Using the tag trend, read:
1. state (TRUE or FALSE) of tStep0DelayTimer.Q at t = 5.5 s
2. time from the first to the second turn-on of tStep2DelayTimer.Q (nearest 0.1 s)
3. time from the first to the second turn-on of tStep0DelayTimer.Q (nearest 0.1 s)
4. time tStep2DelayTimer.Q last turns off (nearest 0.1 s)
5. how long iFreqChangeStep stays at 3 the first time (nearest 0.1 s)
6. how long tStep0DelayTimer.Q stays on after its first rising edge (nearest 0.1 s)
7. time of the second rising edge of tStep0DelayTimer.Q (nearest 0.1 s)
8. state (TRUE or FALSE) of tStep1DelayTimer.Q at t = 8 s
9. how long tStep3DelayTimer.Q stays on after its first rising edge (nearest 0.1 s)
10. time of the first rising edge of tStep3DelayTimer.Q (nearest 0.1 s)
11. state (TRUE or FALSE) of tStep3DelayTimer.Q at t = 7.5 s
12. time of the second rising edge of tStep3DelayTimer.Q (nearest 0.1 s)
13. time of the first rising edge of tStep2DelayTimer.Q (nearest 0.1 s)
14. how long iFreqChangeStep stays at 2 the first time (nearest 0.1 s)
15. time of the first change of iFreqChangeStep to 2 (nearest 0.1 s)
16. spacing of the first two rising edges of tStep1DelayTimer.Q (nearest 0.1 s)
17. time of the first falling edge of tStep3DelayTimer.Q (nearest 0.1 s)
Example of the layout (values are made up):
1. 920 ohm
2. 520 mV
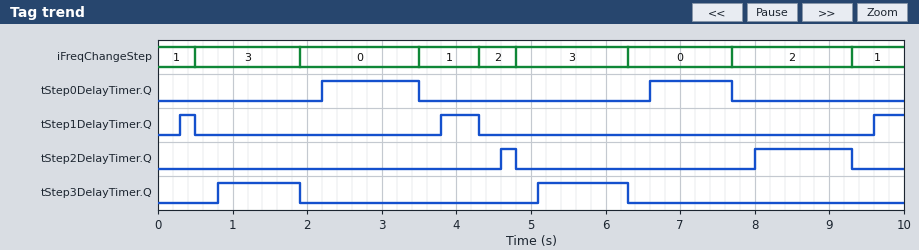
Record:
1. FALSE
2. 3.4 s
3. 4.4 s
4. 9.3 s
5. 1.4 s
6. 1.3 s
7. 6.6 s
8. FALSE
9. 1.1 s
10. 0.8 s
11. FALSE
12. 5.1 s
13. 4.6 s
14. 0.5 s
15. 4.3 s
16. 3.5 s
17. 1.9 s
